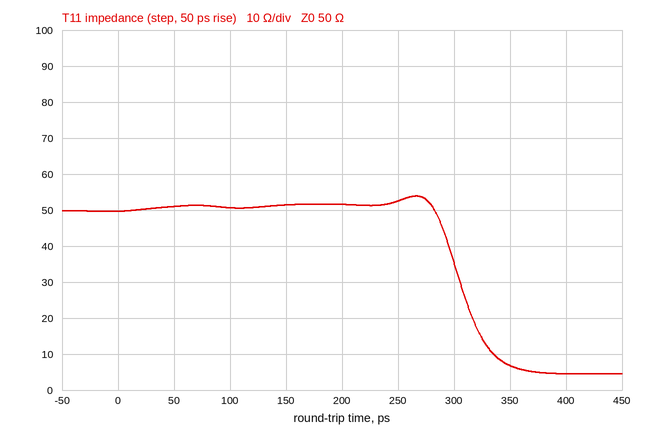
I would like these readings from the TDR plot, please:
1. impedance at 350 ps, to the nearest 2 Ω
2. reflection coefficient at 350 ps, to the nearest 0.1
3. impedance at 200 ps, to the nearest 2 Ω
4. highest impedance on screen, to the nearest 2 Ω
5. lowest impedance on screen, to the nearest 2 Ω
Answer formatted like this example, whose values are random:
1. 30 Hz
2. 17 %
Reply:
1. 6 Ω
2. -0.8
3. 52 Ω
4. 54 Ω
5. 4 Ω
